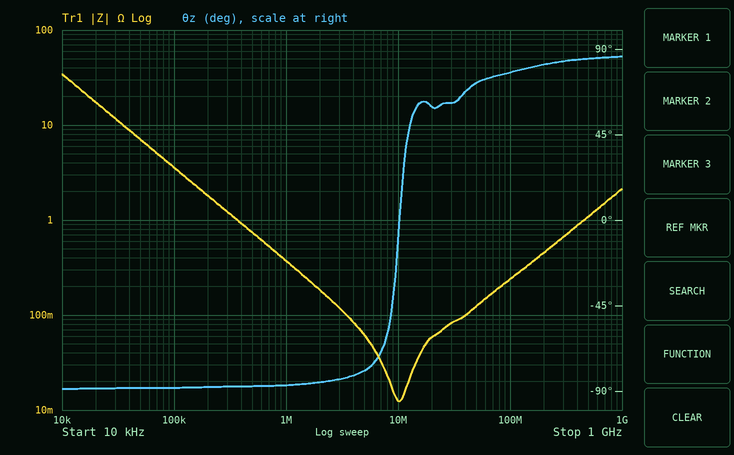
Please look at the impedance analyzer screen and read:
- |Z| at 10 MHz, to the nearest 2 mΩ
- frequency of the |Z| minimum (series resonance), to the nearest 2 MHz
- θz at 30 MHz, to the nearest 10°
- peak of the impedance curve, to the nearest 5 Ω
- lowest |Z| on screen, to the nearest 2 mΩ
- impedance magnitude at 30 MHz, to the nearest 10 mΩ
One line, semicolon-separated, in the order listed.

12 mΩ; 10 MHz; 60°; 35 Ω; 12 mΩ; 80 mΩ
